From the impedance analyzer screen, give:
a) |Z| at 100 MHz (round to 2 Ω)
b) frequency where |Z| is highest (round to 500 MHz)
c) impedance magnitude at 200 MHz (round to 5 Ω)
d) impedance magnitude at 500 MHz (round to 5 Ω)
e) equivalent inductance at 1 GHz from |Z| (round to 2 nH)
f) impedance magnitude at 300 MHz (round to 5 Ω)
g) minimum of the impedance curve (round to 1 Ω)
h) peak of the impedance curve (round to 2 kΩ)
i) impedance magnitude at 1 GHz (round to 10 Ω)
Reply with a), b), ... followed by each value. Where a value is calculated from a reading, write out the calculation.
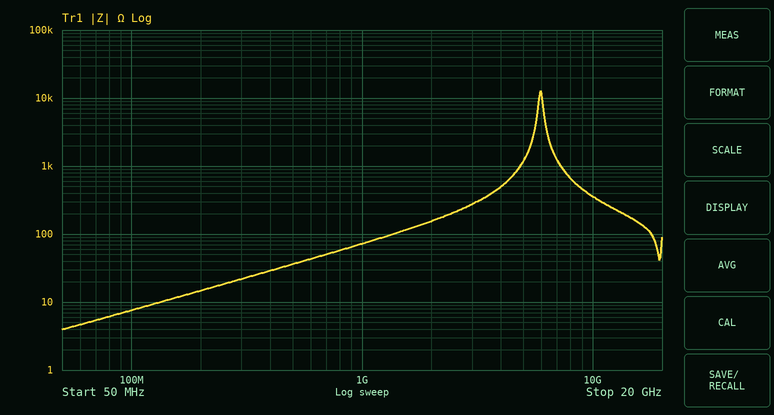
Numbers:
a) 8 Ω
b) 6.0 GHz
c) 15 Ω
d) 35 Ω
e) L = 70 Ω/(2π × 1 GHz) ≈ 11.1 nH, so 12 nH to the nearest 2 nH
f) 20 Ω
g) 4 Ω
h) 12 kΩ
i) 70 Ω
